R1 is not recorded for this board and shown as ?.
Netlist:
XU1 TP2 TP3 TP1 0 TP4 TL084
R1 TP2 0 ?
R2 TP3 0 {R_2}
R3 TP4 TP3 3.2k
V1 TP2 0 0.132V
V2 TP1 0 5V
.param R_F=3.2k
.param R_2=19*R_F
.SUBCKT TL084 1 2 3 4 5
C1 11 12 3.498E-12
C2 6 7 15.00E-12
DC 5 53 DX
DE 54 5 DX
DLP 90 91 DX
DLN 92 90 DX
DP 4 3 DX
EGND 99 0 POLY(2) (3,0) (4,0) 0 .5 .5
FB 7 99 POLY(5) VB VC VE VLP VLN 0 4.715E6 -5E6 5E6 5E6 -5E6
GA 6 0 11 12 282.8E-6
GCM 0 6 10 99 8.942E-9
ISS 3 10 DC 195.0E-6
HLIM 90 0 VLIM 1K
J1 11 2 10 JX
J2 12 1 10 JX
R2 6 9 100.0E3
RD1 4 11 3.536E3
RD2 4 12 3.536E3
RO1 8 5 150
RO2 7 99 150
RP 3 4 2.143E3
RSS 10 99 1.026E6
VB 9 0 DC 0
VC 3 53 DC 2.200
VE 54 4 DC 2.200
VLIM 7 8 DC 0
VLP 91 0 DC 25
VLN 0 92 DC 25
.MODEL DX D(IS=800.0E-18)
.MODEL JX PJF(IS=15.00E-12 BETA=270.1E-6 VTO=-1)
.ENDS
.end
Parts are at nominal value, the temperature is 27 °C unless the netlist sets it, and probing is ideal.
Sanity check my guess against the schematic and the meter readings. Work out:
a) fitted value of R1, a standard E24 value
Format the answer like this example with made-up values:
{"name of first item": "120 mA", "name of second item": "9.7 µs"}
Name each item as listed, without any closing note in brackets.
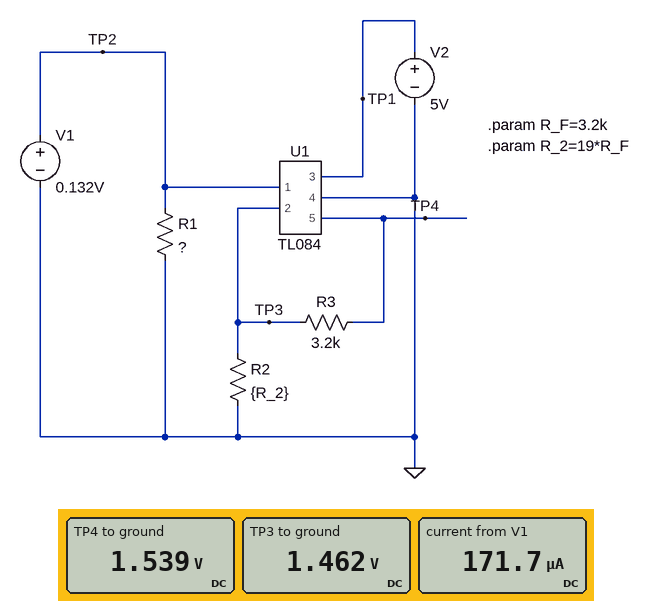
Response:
{"fitted value of R1, a standard E24 value": "510 Ω"}
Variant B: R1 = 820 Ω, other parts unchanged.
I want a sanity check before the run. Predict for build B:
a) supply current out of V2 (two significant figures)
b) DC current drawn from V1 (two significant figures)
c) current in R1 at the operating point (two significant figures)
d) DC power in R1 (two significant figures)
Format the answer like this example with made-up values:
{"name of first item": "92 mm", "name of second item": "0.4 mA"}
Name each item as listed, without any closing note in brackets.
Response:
{"supply current out of V2": "2.5 mA", "DC current drawn from V1": "74 µA", "current in R1 at the operating point": "160 µA", "DC power in R1": "21 µW"}
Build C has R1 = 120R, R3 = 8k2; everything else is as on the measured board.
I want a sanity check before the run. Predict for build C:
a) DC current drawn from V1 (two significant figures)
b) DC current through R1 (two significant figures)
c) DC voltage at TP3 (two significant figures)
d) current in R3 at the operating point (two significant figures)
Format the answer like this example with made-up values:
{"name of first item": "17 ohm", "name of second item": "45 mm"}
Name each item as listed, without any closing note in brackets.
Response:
{"DC current drawn from V1": "1.0 mA", "DC current through R1": "1.1 mA", "DC voltage at TP3": "1.4 V", "current in R3 at the operating point": "22 µA"}
